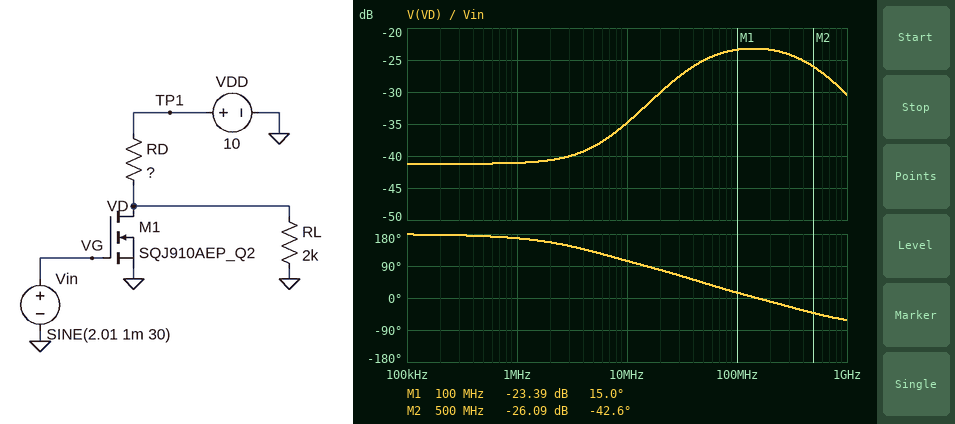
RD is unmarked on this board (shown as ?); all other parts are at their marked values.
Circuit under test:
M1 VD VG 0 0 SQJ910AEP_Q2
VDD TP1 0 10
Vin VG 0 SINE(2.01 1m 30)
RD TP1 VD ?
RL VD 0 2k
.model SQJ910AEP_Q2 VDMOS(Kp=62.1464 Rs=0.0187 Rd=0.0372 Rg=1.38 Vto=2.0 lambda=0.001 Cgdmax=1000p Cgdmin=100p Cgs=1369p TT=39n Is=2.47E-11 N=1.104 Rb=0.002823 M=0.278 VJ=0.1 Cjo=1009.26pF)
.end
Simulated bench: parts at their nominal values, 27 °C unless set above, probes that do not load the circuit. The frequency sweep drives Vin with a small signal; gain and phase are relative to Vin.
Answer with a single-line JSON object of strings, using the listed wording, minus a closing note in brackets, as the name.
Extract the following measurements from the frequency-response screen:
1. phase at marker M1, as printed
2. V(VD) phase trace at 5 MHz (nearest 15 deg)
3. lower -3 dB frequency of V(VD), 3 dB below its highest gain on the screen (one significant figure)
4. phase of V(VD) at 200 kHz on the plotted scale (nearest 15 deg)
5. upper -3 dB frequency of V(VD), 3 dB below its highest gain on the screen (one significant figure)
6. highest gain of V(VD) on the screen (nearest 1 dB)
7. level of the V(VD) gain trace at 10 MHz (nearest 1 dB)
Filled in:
{"phase at marker M1, as printed": "15.0 deg", "V(VD) phase trace at 5 MHz": "135 deg", "lower -3 dB frequency of V(VD), 3 dB below its highest gain on the screen": "40 MHz", "phase of V(VD) at 200 kHz on the plotted scale": "180 deg", "upper -3 dB frequency of V(VD), 3 dB below its highest gain on the screen": "500 MHz", "highest gain of V(VD) on the screen": "-23 dB", "level of the V(VD) gain trace at 10 MHz": "-35 dB"}
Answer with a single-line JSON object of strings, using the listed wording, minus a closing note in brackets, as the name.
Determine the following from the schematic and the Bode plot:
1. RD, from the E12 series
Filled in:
{"RD, from the E12 series": "1.8 kΩ"}
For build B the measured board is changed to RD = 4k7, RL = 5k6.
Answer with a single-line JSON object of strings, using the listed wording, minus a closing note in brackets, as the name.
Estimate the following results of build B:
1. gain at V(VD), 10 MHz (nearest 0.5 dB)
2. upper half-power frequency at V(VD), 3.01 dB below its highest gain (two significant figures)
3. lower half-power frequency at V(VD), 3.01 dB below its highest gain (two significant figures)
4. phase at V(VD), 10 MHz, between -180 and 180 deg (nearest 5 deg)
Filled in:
{"gain at V(VD), 10 MHz": "-36.0 dB", "upper half-power frequency at V(VD), 3.01 dB below its highest gain": "520 MHz", "lower half-power frequency at V(VD), 3.01 dB below its highest gain": "39 MHz", "phase at V(VD), 10 MHz, between -180 and 180 deg": "90 deg"}
